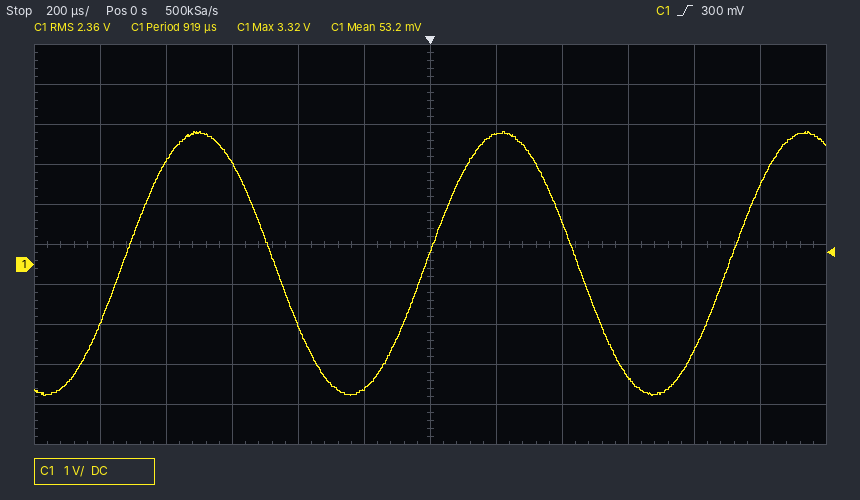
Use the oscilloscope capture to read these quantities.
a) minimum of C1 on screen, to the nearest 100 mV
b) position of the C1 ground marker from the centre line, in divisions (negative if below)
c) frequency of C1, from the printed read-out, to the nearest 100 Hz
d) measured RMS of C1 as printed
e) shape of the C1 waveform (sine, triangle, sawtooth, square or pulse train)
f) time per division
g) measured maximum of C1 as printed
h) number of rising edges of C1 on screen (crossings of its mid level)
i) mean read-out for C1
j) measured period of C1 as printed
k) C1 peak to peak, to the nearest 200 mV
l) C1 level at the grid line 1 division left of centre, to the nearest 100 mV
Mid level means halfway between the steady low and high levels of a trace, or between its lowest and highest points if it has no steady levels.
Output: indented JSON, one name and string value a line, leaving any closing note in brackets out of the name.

{
  "minimum of C1 on screen, to the nearest 100 mV": "-3.3 V",
  "position of the C1 ground marker from the centre line, in divisions": "-0.5 div",
  "frequency of C1, from the printed read-out, to the nearest 100 Hz": "1.1 kHz",
  "measured RMS of C1 as printed": "2.36 V",
  "shape of the C1 waveform": "sine",
  "time per division": "200 µs",
  "measured maximum of C1 as printed": "3.32 V",
  "number of rising edges of C1 on screen": "3",
  "mean read-out for C1": "53.2 mV",
  "measured period of C1 as printed": "919 µs",
  "C1 peak to peak, to the nearest 200 mV": "6.6 V",
  "C1 level at the grid line 1 division left of centre, to the nearest 100 mV": "-3.1 V"
}
